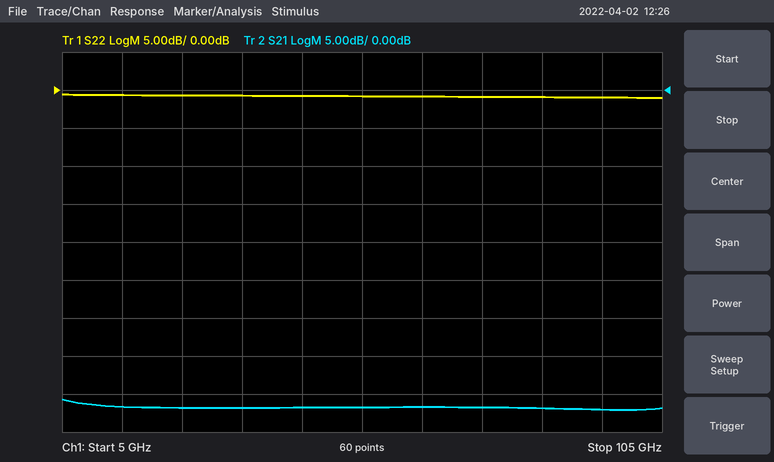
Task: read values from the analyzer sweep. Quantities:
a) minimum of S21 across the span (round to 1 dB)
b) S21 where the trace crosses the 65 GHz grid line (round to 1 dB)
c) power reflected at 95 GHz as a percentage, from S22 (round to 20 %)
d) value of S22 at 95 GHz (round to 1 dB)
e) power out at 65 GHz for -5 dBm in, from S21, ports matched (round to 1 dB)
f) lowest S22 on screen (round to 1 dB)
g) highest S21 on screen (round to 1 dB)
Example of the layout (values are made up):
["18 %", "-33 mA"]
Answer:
["-42 dB", "-42 dB", "80 %", "-1 dB", "-47 dBm", "-1 dB", "-41 dB"]
